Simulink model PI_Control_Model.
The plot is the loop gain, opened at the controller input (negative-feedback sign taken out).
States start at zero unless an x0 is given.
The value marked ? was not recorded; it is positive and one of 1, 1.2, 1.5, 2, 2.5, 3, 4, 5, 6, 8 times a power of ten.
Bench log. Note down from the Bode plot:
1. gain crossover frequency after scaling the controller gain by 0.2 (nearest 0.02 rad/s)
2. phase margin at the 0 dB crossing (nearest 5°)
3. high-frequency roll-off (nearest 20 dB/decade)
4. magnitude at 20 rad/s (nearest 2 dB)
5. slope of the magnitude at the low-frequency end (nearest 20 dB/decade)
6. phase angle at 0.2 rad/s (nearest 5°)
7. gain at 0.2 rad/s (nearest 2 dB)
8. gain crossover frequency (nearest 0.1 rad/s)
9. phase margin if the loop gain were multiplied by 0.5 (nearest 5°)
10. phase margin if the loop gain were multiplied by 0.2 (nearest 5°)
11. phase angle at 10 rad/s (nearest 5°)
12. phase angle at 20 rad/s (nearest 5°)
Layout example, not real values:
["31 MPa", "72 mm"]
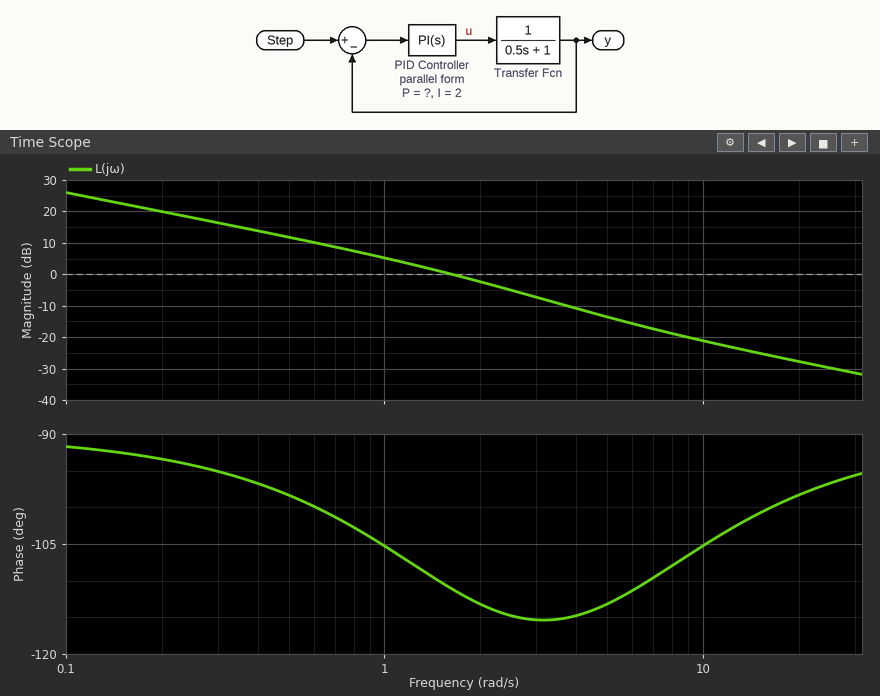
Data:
["0.40 rad/s", "70°", "-20 dB/decade", "-28 dB", "-20 dB/decade", "-95°", "20 dB", "1.6 rad/s", "75°", "85°", "-105°", "-100°"]
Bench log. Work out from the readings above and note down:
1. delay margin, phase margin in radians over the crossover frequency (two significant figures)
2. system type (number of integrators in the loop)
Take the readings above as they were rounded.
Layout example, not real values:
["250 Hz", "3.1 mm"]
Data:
["0.76 s", "1"]
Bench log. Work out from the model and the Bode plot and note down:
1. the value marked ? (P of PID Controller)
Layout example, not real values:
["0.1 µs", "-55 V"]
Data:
["0.4"]
